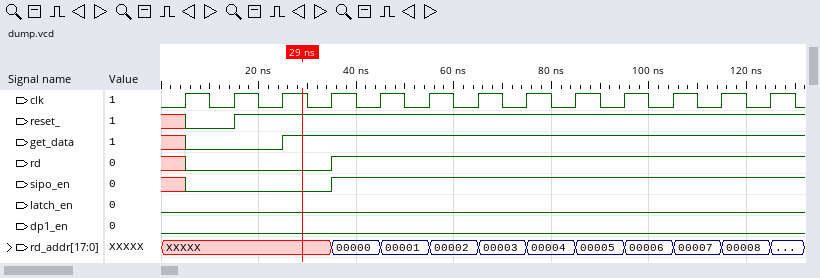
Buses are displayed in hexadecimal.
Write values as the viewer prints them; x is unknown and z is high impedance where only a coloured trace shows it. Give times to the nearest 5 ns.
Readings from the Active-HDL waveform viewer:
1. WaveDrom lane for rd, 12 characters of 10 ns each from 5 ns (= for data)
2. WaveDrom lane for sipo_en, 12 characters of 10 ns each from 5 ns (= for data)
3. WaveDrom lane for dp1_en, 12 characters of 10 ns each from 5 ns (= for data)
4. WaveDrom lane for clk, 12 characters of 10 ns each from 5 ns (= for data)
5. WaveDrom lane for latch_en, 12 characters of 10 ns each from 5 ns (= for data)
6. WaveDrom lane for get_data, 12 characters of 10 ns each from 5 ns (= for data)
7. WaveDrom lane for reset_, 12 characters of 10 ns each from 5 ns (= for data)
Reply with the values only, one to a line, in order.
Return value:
{name: 'rd', wave: '0..1........'}
{name: 'sipo_en', wave: '0..1........'}
{name: 'dp1_en', wave: '0...........'}
{name: 'clk', wave: 'p...........'}
{name: 'latch_en', wave: '0...........'}
{name: 'get_data', wave: '0.1.........'}
{name: 'reset_', wave: '01..........'}
